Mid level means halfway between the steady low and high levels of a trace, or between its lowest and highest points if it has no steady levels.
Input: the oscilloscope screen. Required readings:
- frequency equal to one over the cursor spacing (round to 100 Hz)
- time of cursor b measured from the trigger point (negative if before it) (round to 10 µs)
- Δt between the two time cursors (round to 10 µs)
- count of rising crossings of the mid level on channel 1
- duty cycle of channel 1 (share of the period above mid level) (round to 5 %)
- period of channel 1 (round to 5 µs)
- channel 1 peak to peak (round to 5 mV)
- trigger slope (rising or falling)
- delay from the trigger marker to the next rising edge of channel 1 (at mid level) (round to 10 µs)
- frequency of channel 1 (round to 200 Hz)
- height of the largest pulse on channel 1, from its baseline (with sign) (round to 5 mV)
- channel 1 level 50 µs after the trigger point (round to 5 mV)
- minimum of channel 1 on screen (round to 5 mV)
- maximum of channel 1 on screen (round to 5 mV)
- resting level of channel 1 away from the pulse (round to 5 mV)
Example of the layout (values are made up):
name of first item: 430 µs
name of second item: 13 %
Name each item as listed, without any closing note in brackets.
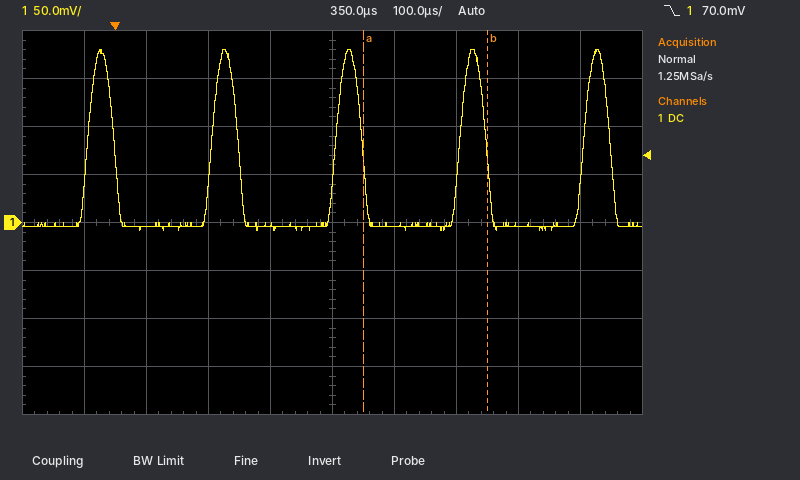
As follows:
frequency equal to one over the cursor spacing: 5.0 kHz
time of cursor b measured from the trigger point (negative if before it): +600 µs
Δt between the two time cursors: 200 µs
count of rising crossings of the mid level on channel 1: 5
duty cycle of channel 1 (share of the period above mid level): 20 %
period of channel 1: 200 µs
channel 1 peak to peak: 190 mV
trigger slope: falling
delay from the trigger marker to the next rising edge of channel 1 (at mid level): 160 µs
frequency of channel 1: 5.0 kHz
height of the largest pulse on channel 1, from its baseline (with sign): +185 mV
channel 1 level 50 µs after the trigger point: -5 mV
minimum of channel 1 on screen: -10 mV
maximum of channel 1 on screen: 180 mV
resting level of channel 1 away from the pulse: -5 mV
